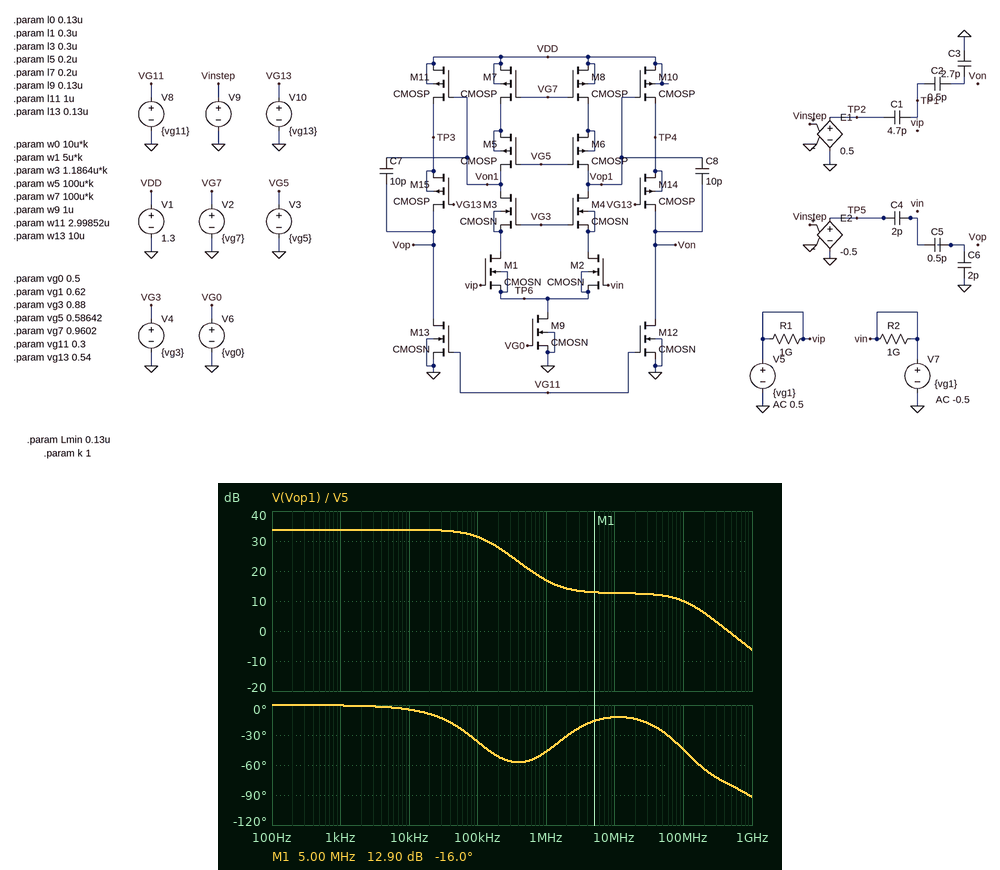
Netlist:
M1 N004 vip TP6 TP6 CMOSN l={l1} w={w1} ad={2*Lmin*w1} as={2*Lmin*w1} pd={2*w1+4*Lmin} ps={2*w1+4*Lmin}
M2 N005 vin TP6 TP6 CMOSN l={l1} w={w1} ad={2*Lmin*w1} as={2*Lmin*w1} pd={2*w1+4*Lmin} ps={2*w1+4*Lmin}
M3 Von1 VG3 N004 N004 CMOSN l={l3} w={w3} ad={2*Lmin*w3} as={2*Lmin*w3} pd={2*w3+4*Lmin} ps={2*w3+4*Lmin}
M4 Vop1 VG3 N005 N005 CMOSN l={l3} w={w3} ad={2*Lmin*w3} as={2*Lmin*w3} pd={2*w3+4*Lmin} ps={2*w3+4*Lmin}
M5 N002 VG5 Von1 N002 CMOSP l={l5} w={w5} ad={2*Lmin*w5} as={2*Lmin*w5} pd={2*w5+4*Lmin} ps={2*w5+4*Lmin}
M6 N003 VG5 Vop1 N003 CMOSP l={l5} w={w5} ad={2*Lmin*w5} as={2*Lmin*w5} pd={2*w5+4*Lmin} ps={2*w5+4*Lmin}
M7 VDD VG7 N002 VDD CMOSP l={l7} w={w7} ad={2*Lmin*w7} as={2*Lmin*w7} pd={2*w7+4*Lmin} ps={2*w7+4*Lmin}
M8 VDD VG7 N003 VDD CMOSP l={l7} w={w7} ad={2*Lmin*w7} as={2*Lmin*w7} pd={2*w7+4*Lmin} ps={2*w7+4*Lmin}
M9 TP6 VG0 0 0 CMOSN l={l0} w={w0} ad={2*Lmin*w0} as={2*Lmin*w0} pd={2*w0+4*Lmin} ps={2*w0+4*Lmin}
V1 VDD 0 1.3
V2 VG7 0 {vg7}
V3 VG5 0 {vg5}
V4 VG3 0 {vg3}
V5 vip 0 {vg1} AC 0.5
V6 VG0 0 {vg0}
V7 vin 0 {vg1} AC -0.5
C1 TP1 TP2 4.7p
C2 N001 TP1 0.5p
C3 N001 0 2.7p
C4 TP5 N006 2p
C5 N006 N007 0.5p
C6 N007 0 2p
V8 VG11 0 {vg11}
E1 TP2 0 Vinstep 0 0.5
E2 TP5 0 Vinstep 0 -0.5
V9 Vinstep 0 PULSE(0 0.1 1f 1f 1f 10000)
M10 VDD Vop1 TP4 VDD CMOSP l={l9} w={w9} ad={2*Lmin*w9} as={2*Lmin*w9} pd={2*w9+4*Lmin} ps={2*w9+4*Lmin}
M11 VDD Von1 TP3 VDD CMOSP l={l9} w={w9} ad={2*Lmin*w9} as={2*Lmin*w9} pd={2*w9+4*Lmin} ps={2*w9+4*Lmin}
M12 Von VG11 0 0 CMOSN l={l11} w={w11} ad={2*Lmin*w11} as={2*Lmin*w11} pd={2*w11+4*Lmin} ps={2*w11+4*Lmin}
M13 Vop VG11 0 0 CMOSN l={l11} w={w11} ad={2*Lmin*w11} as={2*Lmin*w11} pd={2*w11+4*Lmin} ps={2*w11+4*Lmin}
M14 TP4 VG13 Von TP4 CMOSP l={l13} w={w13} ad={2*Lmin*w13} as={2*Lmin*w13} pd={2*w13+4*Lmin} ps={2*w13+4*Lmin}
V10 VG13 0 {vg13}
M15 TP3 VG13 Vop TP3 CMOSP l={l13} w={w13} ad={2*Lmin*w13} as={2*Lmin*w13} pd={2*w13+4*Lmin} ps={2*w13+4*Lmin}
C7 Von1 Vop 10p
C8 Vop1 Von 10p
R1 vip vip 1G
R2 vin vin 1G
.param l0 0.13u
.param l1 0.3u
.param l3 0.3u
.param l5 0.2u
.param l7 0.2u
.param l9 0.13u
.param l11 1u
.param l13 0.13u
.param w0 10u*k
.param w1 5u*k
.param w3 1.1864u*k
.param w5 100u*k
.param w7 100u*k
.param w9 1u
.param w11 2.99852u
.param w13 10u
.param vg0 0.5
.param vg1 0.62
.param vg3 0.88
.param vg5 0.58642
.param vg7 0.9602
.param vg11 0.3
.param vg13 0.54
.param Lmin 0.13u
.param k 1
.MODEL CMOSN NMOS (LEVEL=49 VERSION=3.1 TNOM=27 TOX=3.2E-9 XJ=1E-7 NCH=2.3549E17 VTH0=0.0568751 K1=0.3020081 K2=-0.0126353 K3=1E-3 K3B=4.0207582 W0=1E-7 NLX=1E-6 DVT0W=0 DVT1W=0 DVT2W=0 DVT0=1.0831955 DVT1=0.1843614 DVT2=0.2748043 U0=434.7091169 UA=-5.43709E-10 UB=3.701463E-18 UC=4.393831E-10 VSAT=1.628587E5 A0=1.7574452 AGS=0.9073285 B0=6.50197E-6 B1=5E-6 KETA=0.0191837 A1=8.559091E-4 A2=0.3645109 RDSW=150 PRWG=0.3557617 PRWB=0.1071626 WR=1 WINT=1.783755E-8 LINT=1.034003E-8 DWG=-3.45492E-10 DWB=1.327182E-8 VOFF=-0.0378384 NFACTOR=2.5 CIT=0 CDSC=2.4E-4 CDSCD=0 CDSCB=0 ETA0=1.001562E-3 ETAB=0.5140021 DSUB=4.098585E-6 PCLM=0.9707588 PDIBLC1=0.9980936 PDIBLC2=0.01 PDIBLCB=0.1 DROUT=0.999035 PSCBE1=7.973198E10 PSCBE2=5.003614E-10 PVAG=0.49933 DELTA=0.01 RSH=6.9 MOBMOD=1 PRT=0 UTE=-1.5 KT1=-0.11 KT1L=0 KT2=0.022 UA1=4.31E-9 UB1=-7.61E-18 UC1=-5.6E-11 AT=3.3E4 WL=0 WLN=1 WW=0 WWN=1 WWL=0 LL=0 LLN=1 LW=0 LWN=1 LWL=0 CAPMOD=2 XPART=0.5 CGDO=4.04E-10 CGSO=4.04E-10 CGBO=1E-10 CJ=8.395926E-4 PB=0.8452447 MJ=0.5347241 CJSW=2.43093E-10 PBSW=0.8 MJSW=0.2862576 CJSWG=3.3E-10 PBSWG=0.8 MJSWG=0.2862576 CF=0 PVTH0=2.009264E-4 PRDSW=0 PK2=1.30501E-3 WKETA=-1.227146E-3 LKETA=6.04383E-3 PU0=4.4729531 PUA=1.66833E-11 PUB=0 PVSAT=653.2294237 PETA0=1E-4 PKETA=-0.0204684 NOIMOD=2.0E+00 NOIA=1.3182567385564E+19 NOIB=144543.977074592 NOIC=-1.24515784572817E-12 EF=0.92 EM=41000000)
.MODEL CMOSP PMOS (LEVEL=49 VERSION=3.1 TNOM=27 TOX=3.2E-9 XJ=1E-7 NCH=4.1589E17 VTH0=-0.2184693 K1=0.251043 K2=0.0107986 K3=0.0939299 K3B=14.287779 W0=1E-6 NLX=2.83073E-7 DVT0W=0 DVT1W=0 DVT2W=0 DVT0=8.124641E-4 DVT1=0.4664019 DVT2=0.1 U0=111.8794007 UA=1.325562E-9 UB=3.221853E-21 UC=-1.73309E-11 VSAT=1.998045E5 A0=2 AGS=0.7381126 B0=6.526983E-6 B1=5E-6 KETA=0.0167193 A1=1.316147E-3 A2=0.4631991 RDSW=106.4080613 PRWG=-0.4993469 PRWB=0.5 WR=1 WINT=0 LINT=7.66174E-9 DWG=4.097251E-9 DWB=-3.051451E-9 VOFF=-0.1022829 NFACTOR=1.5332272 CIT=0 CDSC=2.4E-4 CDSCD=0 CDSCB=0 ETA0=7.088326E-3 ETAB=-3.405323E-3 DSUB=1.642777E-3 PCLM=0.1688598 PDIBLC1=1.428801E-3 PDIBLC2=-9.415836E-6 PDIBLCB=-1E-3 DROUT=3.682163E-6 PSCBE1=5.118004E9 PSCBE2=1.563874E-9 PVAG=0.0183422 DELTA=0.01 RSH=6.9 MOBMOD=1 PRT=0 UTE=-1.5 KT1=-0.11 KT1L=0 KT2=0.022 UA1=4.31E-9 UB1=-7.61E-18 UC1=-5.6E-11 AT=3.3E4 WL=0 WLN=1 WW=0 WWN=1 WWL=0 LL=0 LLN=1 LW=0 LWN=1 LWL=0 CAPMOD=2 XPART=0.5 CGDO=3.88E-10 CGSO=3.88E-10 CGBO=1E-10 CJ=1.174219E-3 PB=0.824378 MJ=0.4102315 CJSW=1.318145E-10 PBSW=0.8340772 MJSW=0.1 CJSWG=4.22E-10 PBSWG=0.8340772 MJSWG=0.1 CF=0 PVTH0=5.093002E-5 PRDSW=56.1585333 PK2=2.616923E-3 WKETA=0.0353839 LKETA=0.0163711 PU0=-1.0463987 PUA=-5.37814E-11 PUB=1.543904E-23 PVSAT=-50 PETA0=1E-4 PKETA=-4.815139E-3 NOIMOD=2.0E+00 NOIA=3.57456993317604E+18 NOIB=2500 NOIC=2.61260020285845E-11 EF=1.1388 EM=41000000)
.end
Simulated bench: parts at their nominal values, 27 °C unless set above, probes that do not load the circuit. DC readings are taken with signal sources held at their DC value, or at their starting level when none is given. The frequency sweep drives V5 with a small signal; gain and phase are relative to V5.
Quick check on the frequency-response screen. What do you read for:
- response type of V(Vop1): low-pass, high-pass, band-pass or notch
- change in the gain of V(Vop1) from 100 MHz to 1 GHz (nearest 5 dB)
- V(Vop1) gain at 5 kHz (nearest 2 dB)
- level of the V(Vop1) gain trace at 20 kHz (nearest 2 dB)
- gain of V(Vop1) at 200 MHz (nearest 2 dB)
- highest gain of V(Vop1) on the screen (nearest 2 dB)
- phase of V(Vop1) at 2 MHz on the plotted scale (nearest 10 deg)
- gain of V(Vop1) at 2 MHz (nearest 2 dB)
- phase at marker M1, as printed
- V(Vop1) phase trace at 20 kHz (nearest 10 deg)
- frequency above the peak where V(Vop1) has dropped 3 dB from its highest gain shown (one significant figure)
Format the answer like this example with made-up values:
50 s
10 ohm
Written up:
low-pass
-15 dB
34 dB
34 dB
6 dB
34 dB
-30 deg
14 dB
-16.0 deg
-10 deg
100 kHz
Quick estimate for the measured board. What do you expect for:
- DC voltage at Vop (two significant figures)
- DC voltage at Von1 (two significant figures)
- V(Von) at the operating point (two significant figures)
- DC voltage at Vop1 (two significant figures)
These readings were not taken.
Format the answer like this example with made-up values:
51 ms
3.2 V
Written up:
450 mV
790 mV
450 mV
790 mV
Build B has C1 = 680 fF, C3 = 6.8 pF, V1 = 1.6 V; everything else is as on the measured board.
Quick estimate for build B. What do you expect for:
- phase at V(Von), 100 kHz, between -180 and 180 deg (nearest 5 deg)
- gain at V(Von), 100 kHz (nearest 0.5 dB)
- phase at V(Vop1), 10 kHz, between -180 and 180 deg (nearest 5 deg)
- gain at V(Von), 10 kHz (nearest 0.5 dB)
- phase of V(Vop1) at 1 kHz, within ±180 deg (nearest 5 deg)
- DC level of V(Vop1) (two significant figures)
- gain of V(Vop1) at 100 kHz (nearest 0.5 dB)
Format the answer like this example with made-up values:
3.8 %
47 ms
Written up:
85 deg
-46.5 dB
0 deg
-66.5 dB
0 deg
1.6 V
-23.5 dB
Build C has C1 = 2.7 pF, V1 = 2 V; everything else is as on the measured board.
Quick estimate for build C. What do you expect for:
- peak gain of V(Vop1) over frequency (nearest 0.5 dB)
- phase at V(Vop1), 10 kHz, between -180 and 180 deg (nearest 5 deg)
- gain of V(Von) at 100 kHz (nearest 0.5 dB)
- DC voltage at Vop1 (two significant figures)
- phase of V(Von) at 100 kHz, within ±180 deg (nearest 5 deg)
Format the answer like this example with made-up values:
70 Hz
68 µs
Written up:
-27.5 dB
0 deg
-50.5 dB
2.0 V
85 deg
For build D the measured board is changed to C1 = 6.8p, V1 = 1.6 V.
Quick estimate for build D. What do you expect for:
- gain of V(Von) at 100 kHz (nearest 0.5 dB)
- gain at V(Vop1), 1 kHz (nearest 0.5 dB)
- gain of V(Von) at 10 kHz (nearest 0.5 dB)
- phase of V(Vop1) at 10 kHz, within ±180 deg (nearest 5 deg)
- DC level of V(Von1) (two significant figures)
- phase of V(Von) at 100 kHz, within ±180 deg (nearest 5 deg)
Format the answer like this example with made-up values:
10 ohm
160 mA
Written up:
-46.5 dB
-23.5 dB
-66.5 dB
0 deg
1.6 V
85 deg
